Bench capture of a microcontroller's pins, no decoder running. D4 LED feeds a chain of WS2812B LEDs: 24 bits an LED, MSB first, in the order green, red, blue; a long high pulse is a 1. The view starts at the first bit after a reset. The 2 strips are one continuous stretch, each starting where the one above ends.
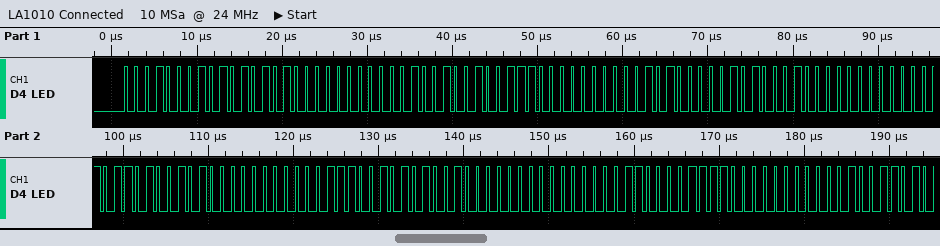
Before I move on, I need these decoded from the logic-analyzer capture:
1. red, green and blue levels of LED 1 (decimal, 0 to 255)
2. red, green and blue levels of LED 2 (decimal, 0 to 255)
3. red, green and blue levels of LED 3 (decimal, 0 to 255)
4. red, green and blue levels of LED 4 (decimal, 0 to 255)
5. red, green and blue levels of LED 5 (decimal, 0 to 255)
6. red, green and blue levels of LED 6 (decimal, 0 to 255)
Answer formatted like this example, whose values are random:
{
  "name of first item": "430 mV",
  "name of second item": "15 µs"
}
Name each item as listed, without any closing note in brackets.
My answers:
{
  "red, green and blue levels of LED 1": "85, 17, 0",
  "red, green and blue levels of LED 2": "78, 18, 0",
  "red, green and blue levels of LED 3": "81, 80, 0",
  "red, green and blue levels of LED 4": "74, 11, 0",
  "red, green and blue levels of LED 5": "82, 57, 0",
  "red, green and blue levels of LED 6": "15, 3, 0"
}
